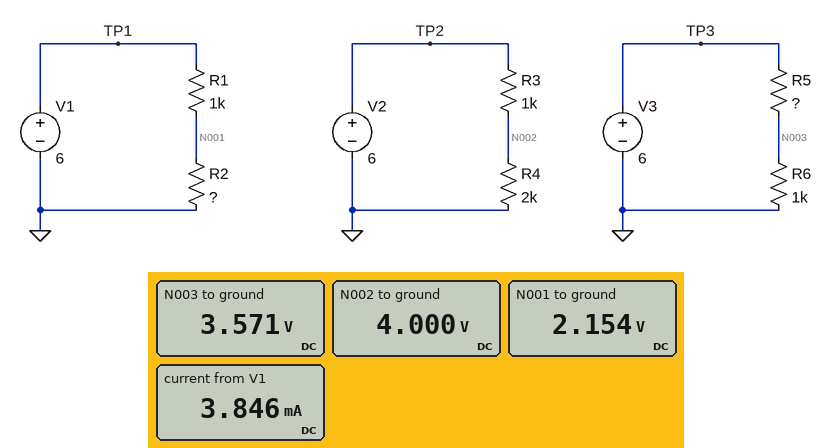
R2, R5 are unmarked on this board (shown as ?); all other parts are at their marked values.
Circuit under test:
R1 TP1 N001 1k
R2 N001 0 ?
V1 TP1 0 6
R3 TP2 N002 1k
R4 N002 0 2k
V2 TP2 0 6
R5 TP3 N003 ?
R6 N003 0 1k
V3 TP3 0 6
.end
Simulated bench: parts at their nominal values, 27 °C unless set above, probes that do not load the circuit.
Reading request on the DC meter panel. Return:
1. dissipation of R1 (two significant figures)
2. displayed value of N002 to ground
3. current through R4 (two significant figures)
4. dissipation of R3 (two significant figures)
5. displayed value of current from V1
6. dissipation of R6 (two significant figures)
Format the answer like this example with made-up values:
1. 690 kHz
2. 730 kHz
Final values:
1. 15 mW
2. 4.000 V
3. 2.0 mA
4. 4.0 mW
5. 3.846 mA
6. 13 mW
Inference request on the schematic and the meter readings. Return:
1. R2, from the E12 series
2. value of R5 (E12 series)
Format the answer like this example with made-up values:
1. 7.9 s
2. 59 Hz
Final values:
1. 560 Ω
2. 680 Ω
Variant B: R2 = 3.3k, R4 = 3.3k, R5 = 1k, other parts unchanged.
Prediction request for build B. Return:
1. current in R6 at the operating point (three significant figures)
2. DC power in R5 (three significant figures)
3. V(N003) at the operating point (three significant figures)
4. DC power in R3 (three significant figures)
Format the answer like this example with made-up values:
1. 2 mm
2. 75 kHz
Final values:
1. 3.00 mA
2. 9.00 mW
3. 3.00 V
4. 1.95 mW
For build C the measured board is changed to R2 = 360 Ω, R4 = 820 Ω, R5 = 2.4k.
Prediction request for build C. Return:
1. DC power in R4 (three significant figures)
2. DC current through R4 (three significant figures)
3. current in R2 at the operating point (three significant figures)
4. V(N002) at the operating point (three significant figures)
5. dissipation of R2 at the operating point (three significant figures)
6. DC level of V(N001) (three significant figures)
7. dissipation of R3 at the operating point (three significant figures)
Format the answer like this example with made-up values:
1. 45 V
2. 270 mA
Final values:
1. 8.91 mW
2. 3.30 mA
3. 4.41 mA
4. 2.70 V
5. 7.01 mW
6. 1.59 V
7. 10.9 mW
